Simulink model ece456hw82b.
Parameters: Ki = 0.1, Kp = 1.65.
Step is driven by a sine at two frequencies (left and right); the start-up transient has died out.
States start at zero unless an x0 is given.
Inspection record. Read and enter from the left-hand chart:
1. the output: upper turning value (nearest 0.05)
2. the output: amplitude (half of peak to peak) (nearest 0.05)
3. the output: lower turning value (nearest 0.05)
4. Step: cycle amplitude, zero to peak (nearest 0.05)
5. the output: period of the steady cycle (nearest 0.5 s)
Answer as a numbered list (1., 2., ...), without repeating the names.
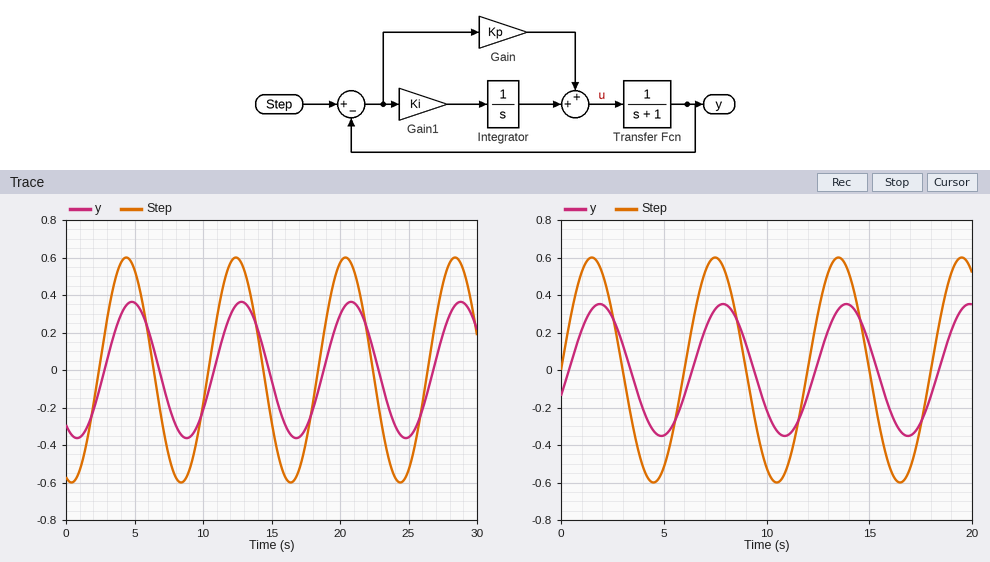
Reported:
1. 0.35
2. 0.35
3. -0.35
4. 0.60
5. 8.0 s
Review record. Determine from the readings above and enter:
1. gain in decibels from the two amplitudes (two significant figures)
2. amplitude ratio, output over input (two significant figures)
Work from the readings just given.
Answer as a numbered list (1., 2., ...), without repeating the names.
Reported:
1. -4.7 dB
2. 0.58
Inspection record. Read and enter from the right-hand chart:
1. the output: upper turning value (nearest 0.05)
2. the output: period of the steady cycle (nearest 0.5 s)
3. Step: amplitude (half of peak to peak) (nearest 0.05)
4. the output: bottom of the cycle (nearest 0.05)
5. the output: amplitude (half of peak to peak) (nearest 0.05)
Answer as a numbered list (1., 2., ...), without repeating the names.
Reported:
1. 0.35
2. 6.0 s
3. 0.60
4. -0.35
5. 0.35
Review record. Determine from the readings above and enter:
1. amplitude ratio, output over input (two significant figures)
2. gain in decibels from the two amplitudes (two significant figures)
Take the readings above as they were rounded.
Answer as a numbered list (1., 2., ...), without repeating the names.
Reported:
1. 0.58
2. -4.7 dB
